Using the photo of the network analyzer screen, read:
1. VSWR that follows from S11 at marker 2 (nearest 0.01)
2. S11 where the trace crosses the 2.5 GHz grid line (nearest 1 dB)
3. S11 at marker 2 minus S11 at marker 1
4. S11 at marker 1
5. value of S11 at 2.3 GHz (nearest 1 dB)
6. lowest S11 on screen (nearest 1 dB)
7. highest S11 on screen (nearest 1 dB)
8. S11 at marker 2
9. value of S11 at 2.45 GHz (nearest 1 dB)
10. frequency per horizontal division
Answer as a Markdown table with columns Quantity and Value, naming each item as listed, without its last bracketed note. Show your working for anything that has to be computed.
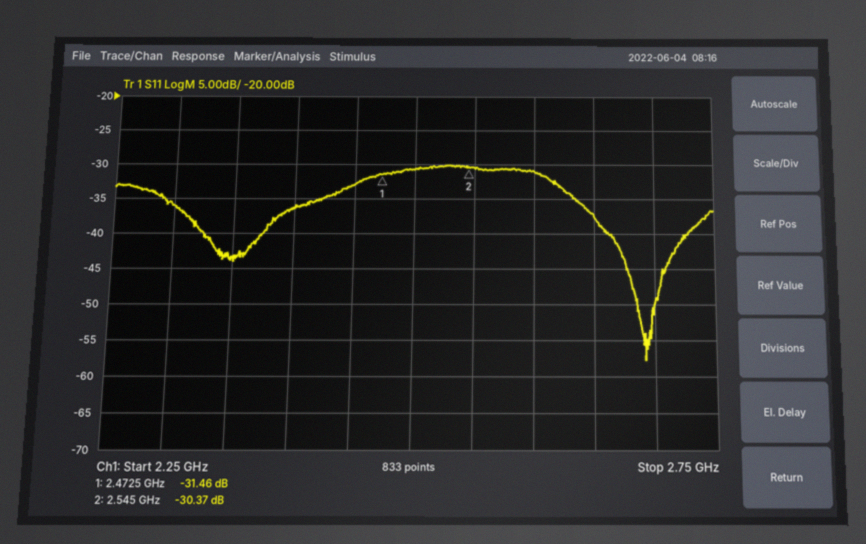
| Quantity | Value |
|---|---|
| VSWR that follows from S11 at marker 2 | (1 + 0.0303)/(1 − 0.0303) ≈ 1.06 |
| S11 where the trace crosses the 2.5 GHz grid line | -31 dB |
| S11 at marker 2 minus S11 at marker 1 | -30.37 − (-31.46) = 1.09 dB |
| S11 at marker 1 | -31.46 dB |
| value of S11 at 2.3 GHz | -36 dB |
| lowest S11 on screen | -58 dB |
| highest S11 on screen | -30 dB |
| S11 at marker 2 | -30.37 dB |
| value of S11 at 2.45 GHz | -33 dB |
| frequency per horizontal division | 50 MHz |
